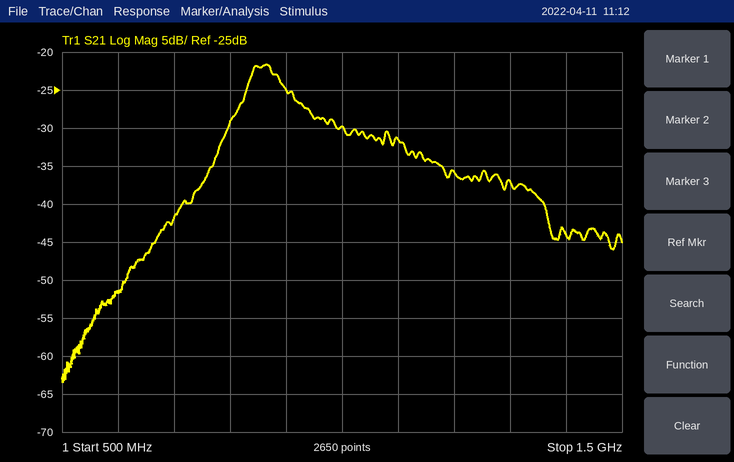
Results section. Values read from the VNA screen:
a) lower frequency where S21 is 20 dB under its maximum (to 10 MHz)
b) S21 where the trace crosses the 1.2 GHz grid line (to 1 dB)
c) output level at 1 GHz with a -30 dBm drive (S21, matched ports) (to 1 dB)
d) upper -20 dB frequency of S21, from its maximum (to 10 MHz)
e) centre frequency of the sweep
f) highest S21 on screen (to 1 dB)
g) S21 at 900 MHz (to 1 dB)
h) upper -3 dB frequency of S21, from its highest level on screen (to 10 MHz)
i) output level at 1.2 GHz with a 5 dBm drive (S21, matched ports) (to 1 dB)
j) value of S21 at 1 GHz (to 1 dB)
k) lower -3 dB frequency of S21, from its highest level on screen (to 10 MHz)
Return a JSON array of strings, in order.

["700 MHz", "-36 dB", "-60 dBm", "1.37 GHz", "1 GHz", "-22 dB", "-25 dB", "900 MHz", "-31 dBm", "-30 dB", "830 MHz"]
